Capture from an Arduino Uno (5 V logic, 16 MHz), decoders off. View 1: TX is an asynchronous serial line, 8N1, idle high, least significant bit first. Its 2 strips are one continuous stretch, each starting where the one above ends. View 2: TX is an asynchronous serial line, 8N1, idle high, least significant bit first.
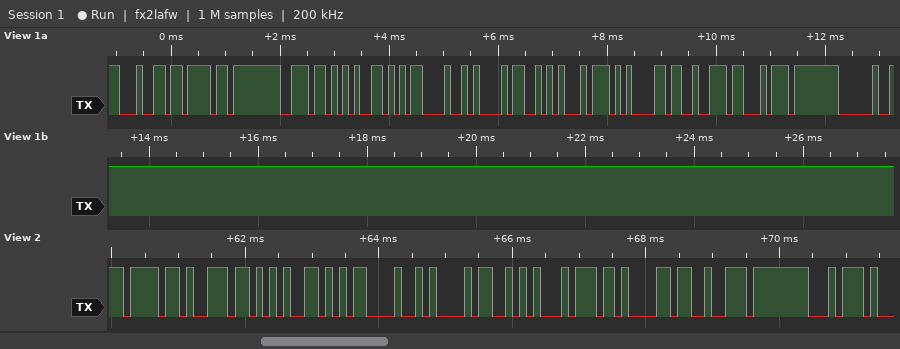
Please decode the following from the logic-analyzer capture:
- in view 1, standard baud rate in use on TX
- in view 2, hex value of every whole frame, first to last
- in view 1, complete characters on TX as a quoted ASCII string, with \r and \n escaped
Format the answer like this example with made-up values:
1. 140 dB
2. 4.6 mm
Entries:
1. 9600 baud
2. 6F 6E 65 0D 0A 53 74 61 72 74
3. "done\r\nStart "
